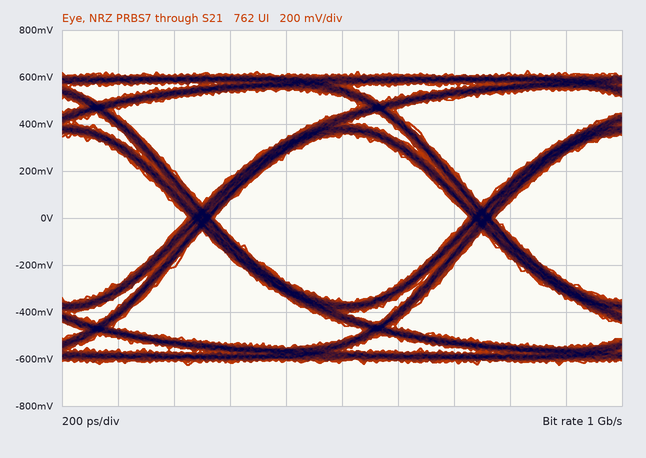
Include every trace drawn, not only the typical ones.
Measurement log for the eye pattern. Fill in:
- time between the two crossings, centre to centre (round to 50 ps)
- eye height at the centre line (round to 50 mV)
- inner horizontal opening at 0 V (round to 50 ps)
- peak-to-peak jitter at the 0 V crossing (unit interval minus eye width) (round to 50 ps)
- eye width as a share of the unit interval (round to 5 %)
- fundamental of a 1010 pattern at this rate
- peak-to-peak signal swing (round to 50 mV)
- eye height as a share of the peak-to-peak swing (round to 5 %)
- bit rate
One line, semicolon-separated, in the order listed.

1.00 ns; 700 mV; 900 ps; 100 ps; 90 %; 500 MHz; 1.25 V; 55 %; 1 Gb/s
